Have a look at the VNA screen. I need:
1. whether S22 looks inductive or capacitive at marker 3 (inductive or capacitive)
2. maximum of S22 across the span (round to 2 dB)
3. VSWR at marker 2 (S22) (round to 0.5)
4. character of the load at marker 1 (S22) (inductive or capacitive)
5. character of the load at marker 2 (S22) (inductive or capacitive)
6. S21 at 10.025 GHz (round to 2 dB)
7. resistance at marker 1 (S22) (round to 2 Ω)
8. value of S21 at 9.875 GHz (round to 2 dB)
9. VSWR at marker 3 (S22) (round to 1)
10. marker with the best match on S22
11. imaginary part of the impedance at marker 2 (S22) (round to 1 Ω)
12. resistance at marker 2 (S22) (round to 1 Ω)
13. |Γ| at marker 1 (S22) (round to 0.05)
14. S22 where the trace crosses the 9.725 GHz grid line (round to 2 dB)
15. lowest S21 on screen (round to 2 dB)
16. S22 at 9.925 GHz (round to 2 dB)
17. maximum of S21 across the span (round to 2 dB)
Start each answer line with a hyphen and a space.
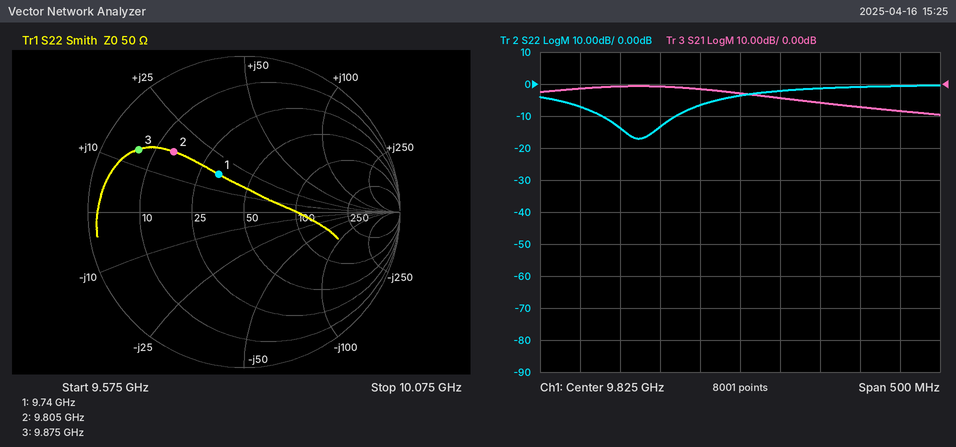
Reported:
- inductive
- 0 dB
- 4.0
- inductive
- inductive
- -8 dB
- 32 Ω
- -4 dB
- 8
- marker 1
- +17 Ω
- 14 Ω
- 0.30
- -14 dB
- -10 dB
- -2 dB
- 0 dB
